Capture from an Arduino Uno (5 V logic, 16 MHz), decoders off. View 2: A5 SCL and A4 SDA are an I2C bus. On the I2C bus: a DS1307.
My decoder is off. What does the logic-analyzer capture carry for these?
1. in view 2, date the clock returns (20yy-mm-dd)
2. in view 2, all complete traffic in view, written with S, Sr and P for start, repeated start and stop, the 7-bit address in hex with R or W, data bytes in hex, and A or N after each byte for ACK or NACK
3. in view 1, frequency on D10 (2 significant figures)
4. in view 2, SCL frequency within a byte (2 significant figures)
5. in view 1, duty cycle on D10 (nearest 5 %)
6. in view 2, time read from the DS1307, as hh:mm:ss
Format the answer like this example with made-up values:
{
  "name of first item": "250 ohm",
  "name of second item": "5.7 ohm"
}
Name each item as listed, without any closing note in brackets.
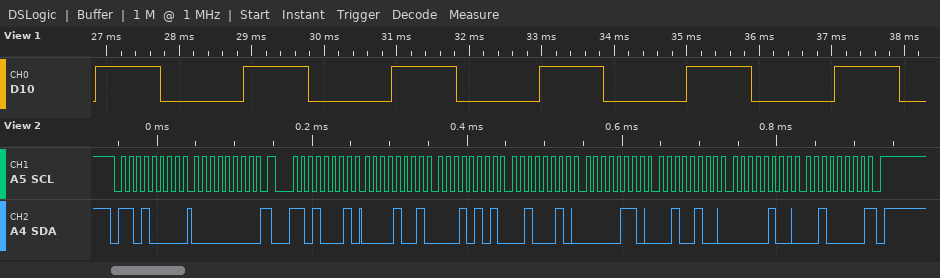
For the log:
{
  "in view 2, date the clock returns": "2020-04-24",
  "in view 2, all complete traffic in view, written with S, Sr and P for start, repeated start and stop, the 7-bit address in hex with R or W, data bytes in hex, and A or N after each byte for ACK or NACK": "S 68W A 00 A Sr 68R A 09 A 15 A 22 A 06 A 24 A 04 A 20 N P",
  "in view 1, frequency on D10": "490 Hz",
  "in view 2, SCL frequency within a byte": "100 kHz",
  "in view 1, duty cycle on D10": "45 %",
  "in view 2, time read from the DS1307, as hh:mm:ss": "22:15:09"
}
